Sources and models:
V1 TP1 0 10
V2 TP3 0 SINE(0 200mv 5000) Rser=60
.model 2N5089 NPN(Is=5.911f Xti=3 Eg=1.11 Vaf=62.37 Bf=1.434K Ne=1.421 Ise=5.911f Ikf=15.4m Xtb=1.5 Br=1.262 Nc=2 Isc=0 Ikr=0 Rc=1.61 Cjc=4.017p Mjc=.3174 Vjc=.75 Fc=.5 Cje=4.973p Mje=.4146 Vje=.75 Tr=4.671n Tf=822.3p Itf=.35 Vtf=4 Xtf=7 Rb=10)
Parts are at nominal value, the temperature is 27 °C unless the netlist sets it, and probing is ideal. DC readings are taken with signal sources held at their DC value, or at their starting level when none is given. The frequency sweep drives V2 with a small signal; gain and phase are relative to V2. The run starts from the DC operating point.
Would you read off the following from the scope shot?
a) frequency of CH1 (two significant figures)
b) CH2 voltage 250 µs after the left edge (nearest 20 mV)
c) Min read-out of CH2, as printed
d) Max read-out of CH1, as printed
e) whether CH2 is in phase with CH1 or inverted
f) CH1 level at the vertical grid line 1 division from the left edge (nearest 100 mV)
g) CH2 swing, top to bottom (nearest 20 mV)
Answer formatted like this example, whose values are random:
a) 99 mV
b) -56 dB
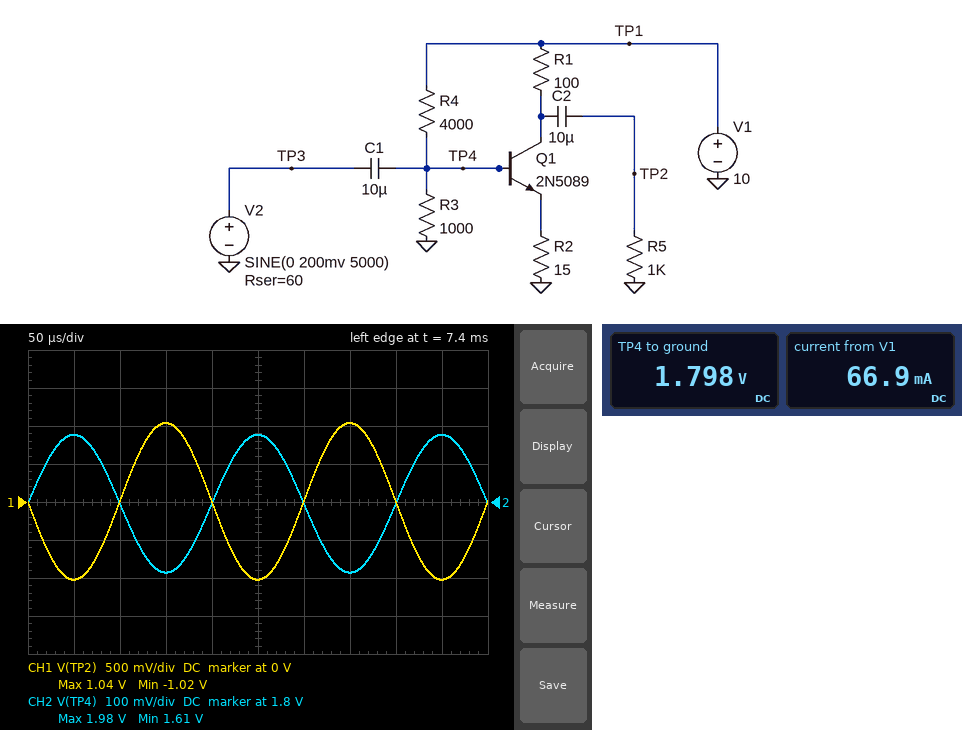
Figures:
a) 5.0 kHz
b) 1.98 V
c) 1.61 V
d) 1.04 V
e) inverted
f) -1.0 V
g) 360 mV
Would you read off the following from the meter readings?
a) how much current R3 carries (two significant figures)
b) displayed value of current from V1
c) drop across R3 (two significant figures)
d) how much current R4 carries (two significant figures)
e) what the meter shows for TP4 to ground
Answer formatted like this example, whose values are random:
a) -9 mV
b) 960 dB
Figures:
a) 1.8 mA
b) 66.9 mA
c) 1.8 V
d) 2.1 mA
e) 1.798 V
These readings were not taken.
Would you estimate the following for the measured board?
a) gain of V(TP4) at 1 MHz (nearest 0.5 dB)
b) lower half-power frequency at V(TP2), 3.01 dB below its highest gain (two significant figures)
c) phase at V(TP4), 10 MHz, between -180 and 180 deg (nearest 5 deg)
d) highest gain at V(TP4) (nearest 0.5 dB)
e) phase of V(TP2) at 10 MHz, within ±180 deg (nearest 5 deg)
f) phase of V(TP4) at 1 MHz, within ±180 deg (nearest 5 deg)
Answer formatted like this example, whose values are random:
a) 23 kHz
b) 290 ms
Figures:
a) -1.0 dB
b) 31 Hz
c) -30 deg
d) -1.0 dB
e) 120 deg
f) -5 deg
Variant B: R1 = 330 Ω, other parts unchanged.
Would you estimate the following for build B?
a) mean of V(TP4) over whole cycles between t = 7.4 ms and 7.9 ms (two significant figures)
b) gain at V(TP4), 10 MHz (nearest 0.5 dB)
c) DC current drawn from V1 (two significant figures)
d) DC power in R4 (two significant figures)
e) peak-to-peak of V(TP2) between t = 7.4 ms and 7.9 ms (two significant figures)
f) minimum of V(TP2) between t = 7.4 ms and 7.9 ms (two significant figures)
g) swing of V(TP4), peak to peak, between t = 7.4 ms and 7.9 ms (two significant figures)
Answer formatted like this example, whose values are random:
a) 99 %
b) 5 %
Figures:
a) 1.2 V
b) -10.5 dB
c) 31 mA
d) 19 mW
e) 2.2 V
f) -320 mV
g) 220 mV
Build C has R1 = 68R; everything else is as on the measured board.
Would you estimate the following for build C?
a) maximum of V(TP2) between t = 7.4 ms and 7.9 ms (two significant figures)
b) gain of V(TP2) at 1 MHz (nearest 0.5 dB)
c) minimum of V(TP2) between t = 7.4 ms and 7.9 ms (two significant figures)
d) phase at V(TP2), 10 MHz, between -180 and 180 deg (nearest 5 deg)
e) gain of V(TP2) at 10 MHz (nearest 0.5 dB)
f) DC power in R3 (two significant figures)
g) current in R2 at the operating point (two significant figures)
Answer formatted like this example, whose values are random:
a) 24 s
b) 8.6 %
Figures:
a) 730 mV
b) 11.0 dB
c) -720 mV
d) 130 deg
e) 7.5 dB
f) 3.3 mW
g) 66 mA
